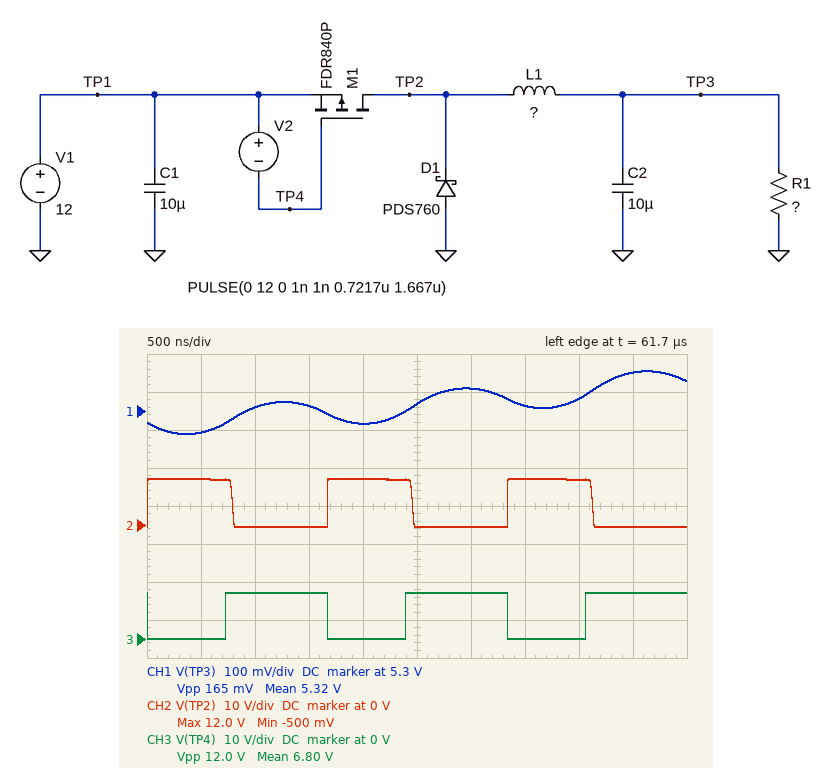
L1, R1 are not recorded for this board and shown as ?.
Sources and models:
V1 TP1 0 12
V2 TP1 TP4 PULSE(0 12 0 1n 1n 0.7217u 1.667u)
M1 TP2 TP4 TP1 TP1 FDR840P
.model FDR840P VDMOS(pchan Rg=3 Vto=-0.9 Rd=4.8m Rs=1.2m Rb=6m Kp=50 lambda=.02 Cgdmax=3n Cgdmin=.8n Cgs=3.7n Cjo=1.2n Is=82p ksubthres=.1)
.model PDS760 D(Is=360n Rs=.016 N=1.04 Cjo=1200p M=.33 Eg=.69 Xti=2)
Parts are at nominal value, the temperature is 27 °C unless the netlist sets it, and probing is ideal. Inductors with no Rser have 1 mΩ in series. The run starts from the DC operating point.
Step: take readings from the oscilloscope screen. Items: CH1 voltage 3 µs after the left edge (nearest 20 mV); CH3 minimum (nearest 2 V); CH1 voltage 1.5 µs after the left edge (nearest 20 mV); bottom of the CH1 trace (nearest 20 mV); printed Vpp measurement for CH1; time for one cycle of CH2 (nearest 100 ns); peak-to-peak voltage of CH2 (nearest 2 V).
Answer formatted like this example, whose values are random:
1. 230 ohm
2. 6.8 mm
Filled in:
1. 5.36 V
2. 0 V
3. 5.32 V
4. 5.24 V
5. 165 mV
6. 1.7 µs
7. 12 V
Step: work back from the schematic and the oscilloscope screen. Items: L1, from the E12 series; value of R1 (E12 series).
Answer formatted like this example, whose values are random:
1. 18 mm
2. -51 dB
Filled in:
1. 1.5 µH
2. 2.2 Ω
